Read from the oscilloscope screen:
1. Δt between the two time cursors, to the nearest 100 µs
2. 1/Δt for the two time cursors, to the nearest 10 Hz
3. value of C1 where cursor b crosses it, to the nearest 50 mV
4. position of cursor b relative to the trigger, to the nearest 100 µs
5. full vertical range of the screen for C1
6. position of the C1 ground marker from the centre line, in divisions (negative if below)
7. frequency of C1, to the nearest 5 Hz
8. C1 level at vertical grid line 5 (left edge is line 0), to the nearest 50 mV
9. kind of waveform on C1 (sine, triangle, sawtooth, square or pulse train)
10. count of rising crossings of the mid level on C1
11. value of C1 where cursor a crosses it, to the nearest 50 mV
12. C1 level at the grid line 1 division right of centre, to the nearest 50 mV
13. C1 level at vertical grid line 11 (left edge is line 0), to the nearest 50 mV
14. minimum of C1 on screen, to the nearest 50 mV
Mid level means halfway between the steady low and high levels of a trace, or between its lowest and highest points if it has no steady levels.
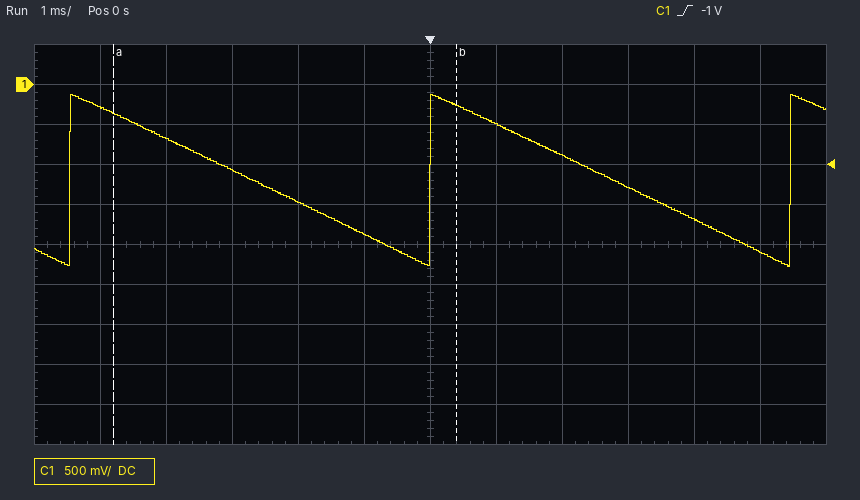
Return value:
5.2 ms
190 Hz
-250 mV
+400 µs
5 V
+4.0 div
185 Hz
-1.85 V
sawtooth
3
-350 mV
-500 mV
-2.10 V
-2.25 V
